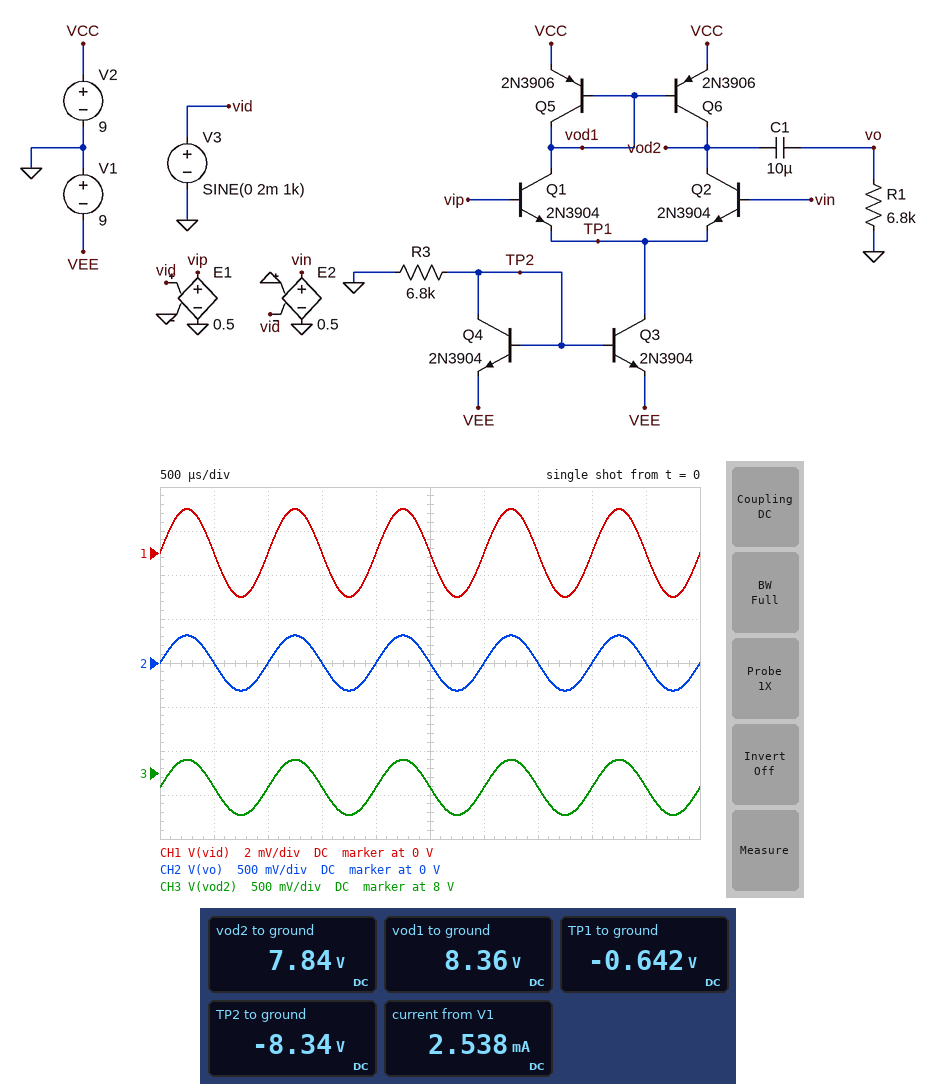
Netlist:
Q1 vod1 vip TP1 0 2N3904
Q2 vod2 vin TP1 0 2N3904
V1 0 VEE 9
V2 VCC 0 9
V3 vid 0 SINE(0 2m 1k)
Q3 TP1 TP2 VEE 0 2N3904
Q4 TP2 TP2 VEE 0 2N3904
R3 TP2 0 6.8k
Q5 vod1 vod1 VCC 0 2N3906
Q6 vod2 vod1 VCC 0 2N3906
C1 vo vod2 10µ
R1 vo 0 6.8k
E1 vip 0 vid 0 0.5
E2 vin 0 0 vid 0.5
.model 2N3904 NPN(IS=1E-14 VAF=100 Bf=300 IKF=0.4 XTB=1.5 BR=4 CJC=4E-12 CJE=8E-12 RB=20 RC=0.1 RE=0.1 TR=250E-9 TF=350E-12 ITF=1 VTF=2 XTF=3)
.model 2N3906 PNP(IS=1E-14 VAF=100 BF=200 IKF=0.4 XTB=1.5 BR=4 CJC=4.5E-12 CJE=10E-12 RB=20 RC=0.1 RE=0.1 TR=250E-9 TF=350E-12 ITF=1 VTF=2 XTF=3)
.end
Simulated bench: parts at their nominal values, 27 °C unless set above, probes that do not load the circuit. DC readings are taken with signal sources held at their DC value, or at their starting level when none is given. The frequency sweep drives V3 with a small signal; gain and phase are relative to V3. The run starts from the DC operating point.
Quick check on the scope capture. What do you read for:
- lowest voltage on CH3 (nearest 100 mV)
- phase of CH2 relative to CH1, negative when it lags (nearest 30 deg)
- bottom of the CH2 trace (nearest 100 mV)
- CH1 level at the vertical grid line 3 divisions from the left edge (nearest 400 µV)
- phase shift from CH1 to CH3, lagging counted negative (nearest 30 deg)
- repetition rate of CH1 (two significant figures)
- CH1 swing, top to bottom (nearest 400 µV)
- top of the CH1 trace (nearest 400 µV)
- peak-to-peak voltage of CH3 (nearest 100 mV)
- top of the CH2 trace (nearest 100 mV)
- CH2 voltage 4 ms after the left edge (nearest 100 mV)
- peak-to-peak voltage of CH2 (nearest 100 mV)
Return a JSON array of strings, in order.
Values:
["7.5 V", "0 deg", "-300 mV", "0 V", "0 deg", "1.0 kHz", "4.0 mV", "2.0 mV", "600 mV", "300 mV", "0 V", "600 mV"]
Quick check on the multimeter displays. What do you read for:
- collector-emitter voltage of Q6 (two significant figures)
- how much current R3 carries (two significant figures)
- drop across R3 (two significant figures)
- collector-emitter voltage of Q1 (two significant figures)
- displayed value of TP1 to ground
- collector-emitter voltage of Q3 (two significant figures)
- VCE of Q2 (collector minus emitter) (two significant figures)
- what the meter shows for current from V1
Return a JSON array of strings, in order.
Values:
["-1.2 V", "1.2 mA", "8.3 V", "9.0 V", "-0.642 V", "8.4 V", "8.5 V", "2.538 mA"]
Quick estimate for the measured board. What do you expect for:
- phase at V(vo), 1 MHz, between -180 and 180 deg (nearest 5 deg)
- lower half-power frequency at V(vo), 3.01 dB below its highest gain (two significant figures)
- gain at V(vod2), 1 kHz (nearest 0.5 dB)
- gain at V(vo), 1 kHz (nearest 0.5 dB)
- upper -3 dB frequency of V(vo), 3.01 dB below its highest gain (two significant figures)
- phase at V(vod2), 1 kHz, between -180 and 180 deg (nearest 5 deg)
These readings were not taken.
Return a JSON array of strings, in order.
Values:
["-25 deg", "180 mHz", "44.0 dB", "44.0 dB", "2.1 MHz", "0 deg"]
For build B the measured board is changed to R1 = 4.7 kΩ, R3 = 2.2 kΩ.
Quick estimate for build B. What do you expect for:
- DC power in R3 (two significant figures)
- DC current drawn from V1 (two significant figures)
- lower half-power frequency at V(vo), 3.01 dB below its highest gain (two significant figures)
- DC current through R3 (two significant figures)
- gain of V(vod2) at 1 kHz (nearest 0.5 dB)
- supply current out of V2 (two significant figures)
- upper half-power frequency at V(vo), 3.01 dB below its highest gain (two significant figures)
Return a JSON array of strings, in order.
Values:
["31 mW", "7.8 mA", "520 mHz", "3.8 mA", "49.5 dB", "4.0 mA", "2.2 MHz"]
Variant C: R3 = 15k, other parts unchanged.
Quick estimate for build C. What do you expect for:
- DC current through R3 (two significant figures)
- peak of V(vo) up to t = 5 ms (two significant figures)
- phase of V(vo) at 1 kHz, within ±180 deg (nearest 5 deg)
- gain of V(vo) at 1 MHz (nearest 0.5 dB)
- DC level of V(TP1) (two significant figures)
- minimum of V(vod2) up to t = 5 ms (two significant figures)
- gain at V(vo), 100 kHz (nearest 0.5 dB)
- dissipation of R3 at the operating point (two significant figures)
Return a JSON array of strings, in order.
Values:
["560 µA", "150 mV", "0 deg", "36.5 dB", "-620 mV", "7.7 V", "37.5 dB", "4.7 mW"]
